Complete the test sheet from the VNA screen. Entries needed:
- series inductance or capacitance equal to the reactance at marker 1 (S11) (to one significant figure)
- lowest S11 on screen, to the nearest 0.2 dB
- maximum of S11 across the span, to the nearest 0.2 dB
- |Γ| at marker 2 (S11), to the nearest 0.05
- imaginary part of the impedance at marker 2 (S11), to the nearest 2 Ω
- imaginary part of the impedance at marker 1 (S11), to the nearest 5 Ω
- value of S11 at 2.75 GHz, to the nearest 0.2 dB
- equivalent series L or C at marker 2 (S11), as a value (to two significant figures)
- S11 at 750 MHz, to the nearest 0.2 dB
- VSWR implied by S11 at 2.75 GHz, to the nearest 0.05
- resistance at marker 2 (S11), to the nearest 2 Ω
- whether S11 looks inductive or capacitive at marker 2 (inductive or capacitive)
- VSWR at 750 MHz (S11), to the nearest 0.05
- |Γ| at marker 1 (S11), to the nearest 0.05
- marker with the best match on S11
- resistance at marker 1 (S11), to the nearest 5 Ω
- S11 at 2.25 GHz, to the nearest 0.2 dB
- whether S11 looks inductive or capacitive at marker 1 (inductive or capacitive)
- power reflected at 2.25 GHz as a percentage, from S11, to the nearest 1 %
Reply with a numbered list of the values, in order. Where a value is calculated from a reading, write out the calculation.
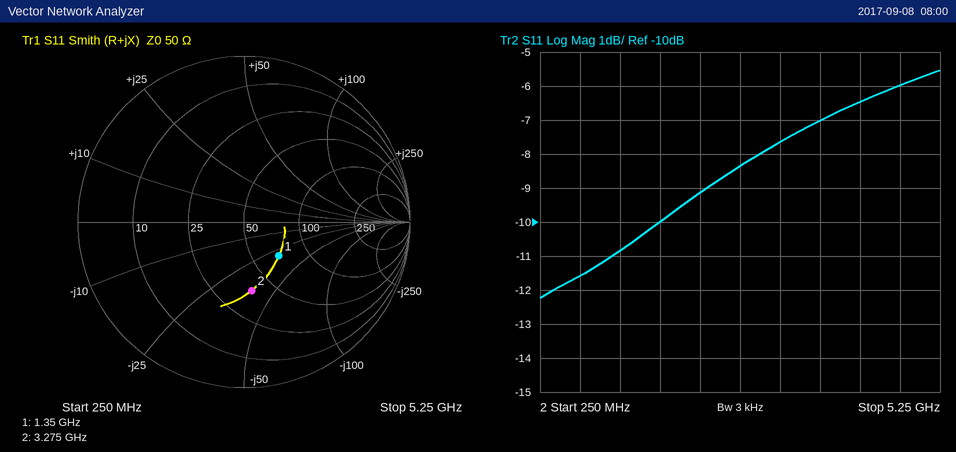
1. C = 1/(2π × 1.35 GHz × 30 Ω) ≈ 4 pF
2. -12.2 dB
3. -5.6 dB
4. 0.40
5. -38 Ω
6. -30 Ω
7. -8.4 dB
8. C = 1/(2π × 3.275 GHz × 38 Ω) ≈ 1.3 pF
9. -11.6 dB
10. |Γ| = 10^(-8.4/20) = 0.3802; VSWR = (1 + 0.3802)/(1 − 0.3802) ≈ 2.23, so 2.25 to the nearest 0.05
11. 38 Ω
12. capacitive
13. |Γ| = 10^(-11.6/20) = 0.2630; VSWR = (1 + 0.2630)/(1 − 0.2630) ≈ 1.71, so 1.70 to the nearest 0.05
14. 0.30
15. marker 1
16. 70 Ω
17. -9.2 dB
18. capacitive
19. 10^(-9.2/10) ≈ 12 %
